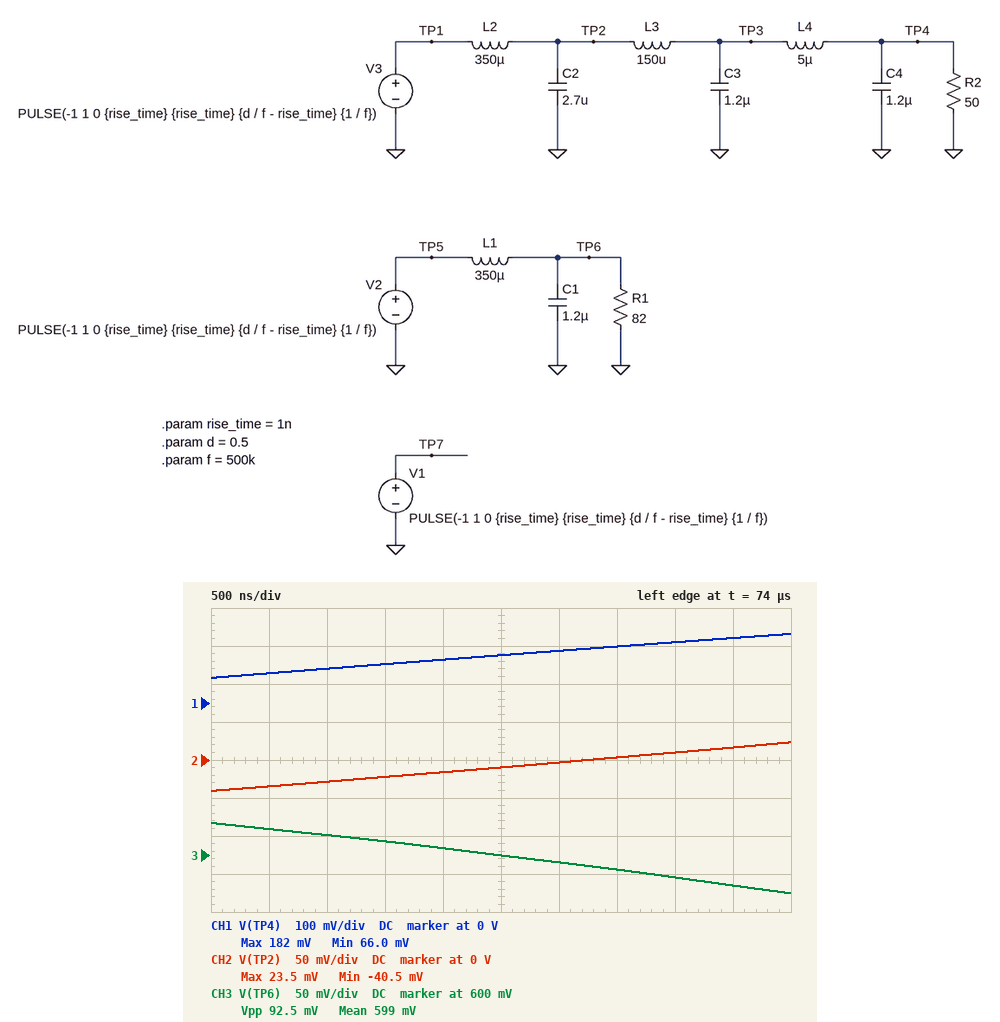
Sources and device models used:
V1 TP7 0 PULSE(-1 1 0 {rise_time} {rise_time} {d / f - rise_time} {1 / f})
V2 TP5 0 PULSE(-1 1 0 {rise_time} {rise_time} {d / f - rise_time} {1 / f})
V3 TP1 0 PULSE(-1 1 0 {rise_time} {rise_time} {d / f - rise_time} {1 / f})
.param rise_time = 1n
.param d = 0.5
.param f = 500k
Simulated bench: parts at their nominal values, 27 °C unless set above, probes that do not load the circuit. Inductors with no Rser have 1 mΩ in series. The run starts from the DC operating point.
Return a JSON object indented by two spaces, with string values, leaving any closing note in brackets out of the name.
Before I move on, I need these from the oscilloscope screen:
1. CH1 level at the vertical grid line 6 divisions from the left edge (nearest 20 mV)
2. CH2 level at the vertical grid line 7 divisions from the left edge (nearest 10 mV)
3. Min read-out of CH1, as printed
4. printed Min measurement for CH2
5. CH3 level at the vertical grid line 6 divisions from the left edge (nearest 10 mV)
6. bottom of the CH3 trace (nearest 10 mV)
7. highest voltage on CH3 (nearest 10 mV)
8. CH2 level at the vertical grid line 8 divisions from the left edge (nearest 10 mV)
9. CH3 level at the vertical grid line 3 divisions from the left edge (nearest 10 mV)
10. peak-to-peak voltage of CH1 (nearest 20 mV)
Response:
{
  "CH1 level at the vertical grid line 6 divisions from the left edge": "140 mV",
  "CH2 level at the vertical grid line 7 divisions from the left edge": "0 V",
  "Min read-out of CH1, as printed": "66.0 mV",
  "printed Min measurement for CH2": "-40.5 mV",
  "CH3 level at the vertical grid line 6 divisions from the left edge": "590 mV",
  "bottom of the CH3 trace": "550 mV",
  "highest voltage on CH3": "640 mV",
  "CH2 level at the vertical grid line 8 divisions from the left edge": "10 mV",
  "CH3 level at the vertical grid line 3 divisions from the left edge": "620 mV",
  "peak-to-peak voltage of CH1": "120 mV"
}
